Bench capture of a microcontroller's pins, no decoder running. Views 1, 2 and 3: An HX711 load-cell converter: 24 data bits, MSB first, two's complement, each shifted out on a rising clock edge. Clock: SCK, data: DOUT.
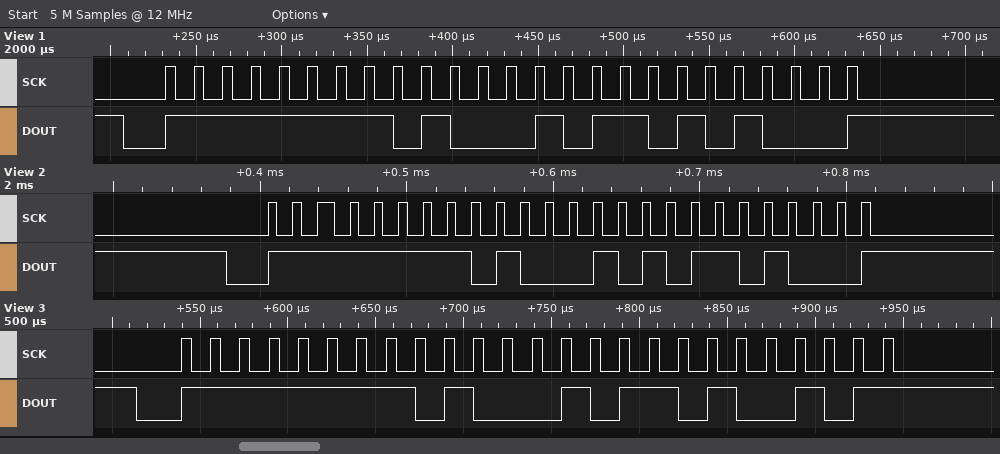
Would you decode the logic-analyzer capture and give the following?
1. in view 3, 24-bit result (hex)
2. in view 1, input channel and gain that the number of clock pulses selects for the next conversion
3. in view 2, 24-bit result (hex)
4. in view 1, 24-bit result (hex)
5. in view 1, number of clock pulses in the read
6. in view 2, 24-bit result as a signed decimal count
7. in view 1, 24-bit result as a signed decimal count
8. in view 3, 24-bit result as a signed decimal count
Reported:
0xFF45A5
channel A, gain 128
0xFF4568
0xFF45A8
25
-47768
-47704
-47707
